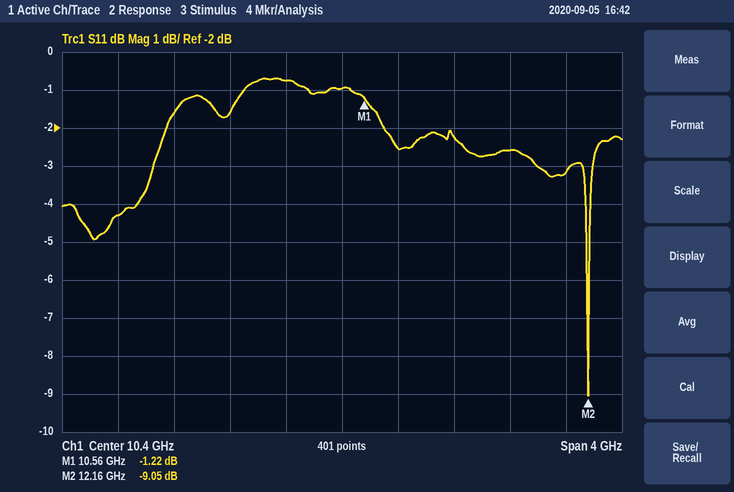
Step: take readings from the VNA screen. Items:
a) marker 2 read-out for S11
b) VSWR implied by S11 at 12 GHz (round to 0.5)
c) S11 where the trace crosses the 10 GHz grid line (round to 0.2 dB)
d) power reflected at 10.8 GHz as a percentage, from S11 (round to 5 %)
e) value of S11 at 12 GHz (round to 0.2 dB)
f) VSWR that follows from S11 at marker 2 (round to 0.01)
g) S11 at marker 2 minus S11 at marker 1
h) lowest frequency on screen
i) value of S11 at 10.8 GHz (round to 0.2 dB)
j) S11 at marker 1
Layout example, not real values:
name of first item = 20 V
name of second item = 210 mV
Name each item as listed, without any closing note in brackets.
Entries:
marker 2 read-out for S11 = -9.05 dB
VSWR implied by S11 at 12 GHz = 5.5
S11 where the trace crosses the 10 GHz grid line = -0.8 dB
power reflected at 10.8 GHz as a percentage, from S11 = 55 %
value of S11 at 12 GHz = -3.2 dB
VSWR that follows from S11 at marker 2 = 2.09
S11 at marker 2 minus S11 at marker 1 = -7.83 dB
lowest frequency on screen = 8.4 GHz
value of S11 at 10.8 GHz = -2.6 dB
S11 at marker 1 = -1.22 dB
